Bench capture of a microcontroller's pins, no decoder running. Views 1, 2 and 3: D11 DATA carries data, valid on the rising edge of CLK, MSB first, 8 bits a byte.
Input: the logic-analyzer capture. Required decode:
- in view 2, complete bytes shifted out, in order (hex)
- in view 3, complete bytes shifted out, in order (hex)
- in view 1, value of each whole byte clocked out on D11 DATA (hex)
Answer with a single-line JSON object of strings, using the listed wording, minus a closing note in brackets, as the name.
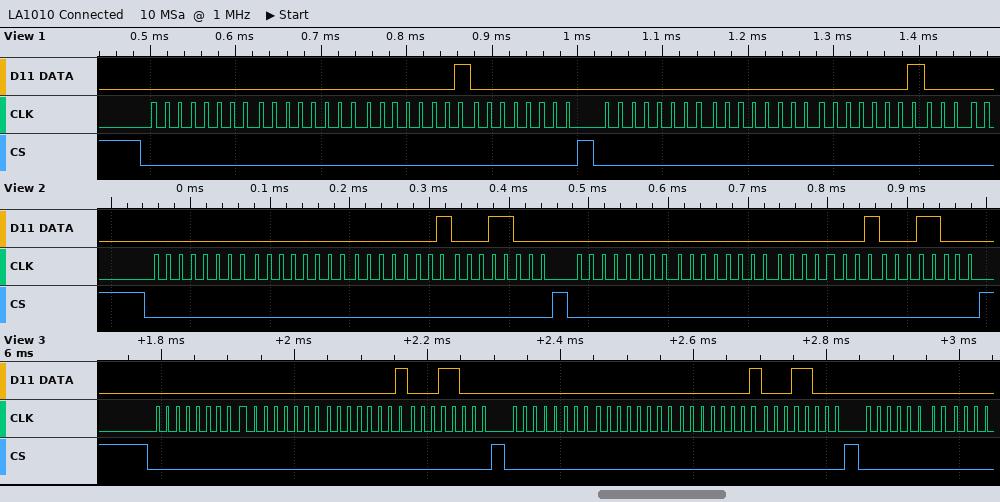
{"in view 2, complete bytes shifted out, in order": "00 00 01 18 00 00 01 18", "in view 3, complete bytes shifted out, in order": "0x00 0x00 0x01 0x18 0x00 0x00 0x01 0x18 0x00", "in view 1, value of each whole byte clocked out on D11 DATA": "00 00 01 00 00 00 01"}
